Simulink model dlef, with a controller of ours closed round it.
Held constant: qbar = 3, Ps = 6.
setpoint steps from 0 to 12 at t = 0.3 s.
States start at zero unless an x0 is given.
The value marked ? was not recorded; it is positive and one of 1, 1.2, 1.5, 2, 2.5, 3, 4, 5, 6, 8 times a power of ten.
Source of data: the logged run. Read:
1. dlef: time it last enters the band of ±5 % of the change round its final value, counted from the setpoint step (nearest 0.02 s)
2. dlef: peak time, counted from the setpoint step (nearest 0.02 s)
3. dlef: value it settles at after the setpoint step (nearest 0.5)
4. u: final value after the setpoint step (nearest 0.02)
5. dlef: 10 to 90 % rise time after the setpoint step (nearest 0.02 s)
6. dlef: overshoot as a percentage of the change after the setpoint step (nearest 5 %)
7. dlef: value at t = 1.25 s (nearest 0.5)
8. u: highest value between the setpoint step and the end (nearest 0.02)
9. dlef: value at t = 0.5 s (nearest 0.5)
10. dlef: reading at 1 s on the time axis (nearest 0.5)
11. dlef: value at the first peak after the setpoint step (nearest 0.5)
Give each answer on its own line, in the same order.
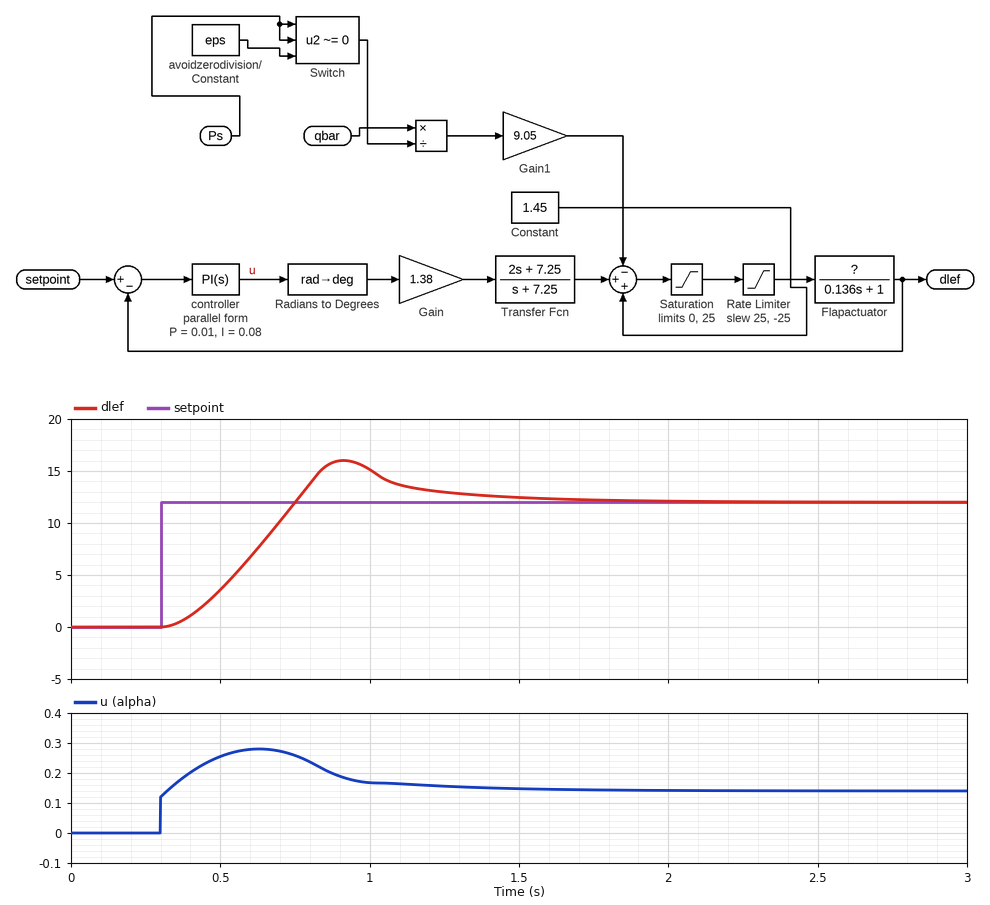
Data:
1.10 s
0.62 s
12.0
0.14
0.32 s
35 %
13.0
0.28
3.5
15.0
16.0
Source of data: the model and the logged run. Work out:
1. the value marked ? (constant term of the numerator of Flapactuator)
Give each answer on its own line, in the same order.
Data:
1.5
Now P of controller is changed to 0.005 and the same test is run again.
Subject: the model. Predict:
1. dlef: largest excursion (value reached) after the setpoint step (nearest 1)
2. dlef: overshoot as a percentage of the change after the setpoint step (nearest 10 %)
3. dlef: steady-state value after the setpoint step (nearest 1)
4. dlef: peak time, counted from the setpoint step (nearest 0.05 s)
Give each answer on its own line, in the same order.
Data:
17
40 %
12
0.65 s
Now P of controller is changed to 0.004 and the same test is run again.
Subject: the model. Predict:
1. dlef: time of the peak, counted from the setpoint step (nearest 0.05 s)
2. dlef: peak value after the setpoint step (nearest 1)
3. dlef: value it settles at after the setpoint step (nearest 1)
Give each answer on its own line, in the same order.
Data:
0.65 s
17
12
